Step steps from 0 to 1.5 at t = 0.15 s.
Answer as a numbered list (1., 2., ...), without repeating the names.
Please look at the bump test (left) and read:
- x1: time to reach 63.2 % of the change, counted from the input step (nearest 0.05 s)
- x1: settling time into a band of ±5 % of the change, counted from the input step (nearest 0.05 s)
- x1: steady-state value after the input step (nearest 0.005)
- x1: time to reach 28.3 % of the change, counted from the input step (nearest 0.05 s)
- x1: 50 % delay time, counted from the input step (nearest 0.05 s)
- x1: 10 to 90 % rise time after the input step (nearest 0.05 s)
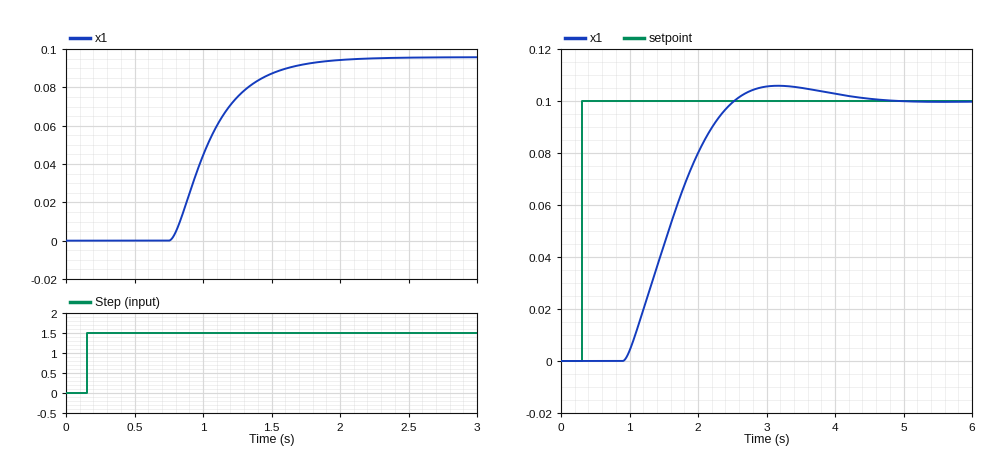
1. 0.95 s
2. 1.50 s
3. 0.095
4. 0.75 s
5. 0.85 s
6. 0.65 s
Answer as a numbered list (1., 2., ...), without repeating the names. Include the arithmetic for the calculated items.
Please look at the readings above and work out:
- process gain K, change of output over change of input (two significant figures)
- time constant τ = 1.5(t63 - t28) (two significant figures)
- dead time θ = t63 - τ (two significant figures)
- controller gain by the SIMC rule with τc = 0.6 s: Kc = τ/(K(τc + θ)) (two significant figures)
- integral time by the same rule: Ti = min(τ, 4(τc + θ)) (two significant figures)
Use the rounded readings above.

1. (0.095 - 0) / 1.5 = 0.063
2. 1.5 × (0.95 - 0.75) = 0.30 s
3. 0.95 - 0.3 = 0.65 s
4. 0.3 / (0.063 × (0.6 + 0.65)) = 3.8
5. min(0.3, 4 × (0.6 + 0.65)) = 0.30 s
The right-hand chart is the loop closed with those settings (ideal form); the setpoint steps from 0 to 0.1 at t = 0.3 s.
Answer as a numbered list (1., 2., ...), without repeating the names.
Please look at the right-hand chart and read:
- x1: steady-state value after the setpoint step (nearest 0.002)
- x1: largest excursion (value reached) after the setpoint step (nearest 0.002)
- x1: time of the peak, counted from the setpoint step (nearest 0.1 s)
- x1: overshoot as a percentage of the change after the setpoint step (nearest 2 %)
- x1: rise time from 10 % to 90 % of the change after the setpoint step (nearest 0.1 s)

1. 0.100
2. 0.106
3. 2.9 s
4. 6 %
5. 1.1 s
